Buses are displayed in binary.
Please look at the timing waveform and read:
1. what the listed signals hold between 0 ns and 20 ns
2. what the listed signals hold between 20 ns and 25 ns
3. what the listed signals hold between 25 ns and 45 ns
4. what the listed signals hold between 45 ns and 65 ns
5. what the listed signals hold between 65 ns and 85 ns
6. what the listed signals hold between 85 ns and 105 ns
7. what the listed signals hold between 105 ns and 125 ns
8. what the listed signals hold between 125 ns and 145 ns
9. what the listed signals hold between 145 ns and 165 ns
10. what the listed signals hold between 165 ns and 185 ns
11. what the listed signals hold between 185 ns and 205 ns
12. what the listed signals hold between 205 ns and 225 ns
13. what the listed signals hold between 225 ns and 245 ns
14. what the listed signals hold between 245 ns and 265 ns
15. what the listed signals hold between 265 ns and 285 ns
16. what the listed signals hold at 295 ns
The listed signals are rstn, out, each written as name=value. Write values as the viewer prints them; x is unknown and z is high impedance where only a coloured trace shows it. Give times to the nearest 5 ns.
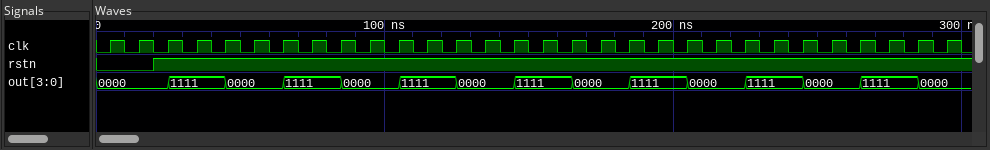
rstn=0, out=0000
rstn=1, out=0000
rstn=1, out=1111
rstn=1, out=0000
rstn=1, out=1111
rstn=1, out=0000
rstn=1, out=1111
rstn=1, out=0000
rstn=1, out=1111
rstn=1, out=0000
rstn=1, out=1111
rstn=1, out=0000
rstn=1, out=1111
rstn=1, out=0000
rstn=1, out=1111
rstn=1, out=0000
